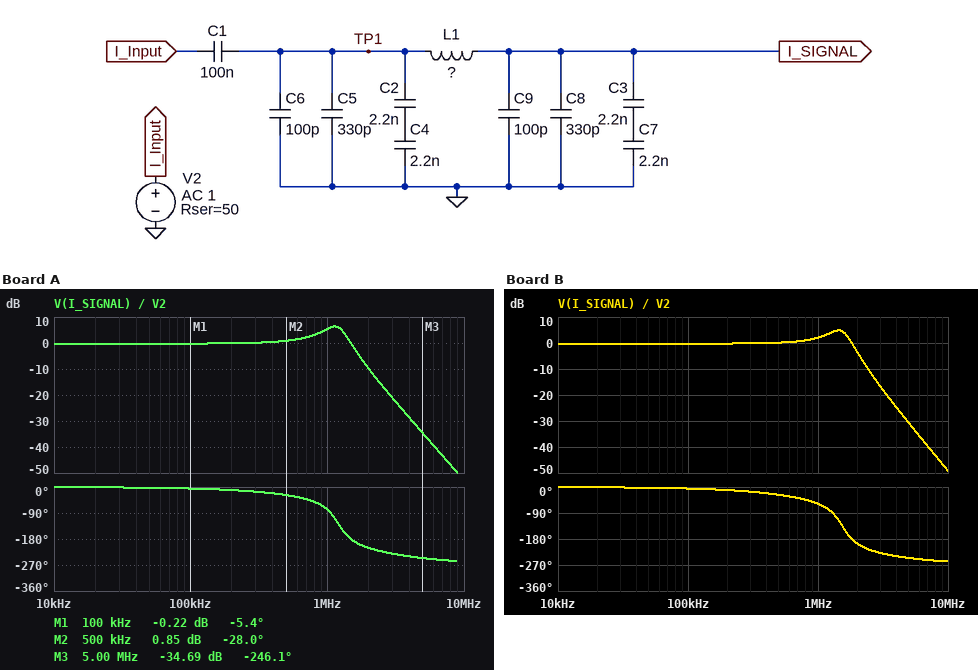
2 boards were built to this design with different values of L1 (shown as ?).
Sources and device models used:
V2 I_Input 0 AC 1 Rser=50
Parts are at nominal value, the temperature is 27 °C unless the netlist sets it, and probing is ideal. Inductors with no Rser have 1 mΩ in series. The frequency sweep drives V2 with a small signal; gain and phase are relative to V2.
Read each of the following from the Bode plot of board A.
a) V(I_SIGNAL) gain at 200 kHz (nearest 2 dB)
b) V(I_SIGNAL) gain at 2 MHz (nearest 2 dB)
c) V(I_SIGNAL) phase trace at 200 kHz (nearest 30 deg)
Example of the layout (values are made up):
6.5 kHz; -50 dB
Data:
0 dB; -10 dB; 0 deg
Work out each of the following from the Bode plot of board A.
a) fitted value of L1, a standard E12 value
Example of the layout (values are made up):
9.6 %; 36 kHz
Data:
15 µH
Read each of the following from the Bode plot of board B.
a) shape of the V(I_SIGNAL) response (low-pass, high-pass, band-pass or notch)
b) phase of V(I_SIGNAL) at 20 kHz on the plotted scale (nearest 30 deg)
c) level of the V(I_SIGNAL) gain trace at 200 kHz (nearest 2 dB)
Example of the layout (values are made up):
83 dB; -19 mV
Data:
low-pass; 0 deg; 0 dB
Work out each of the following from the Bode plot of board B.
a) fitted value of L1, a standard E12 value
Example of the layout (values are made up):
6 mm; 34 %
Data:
10 µH
